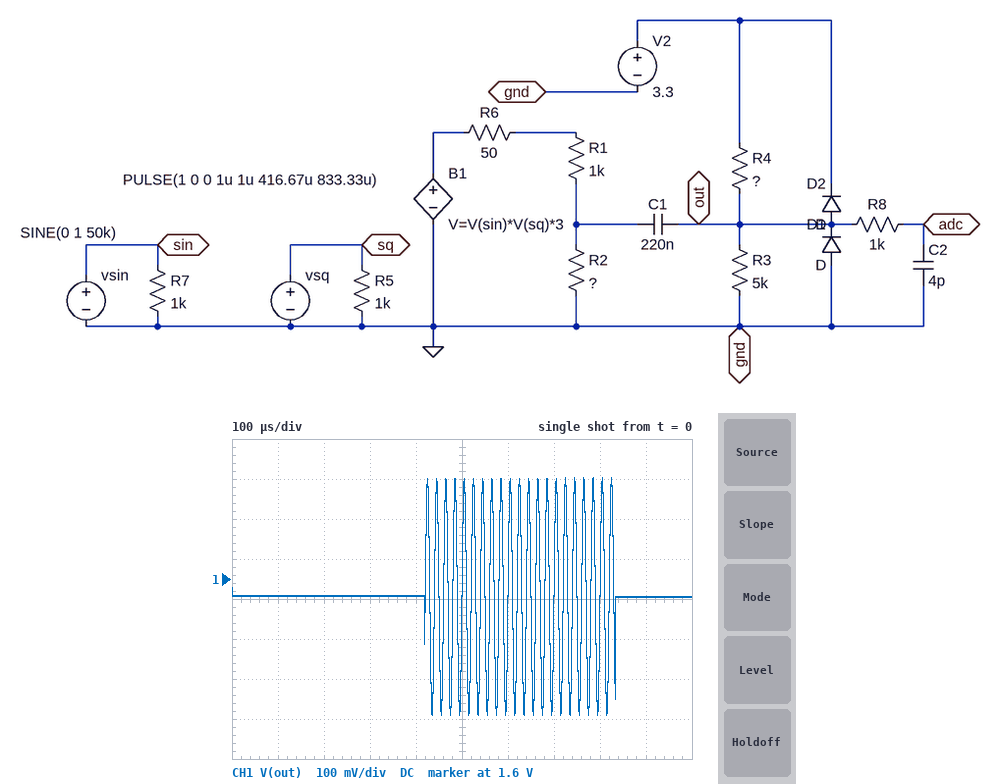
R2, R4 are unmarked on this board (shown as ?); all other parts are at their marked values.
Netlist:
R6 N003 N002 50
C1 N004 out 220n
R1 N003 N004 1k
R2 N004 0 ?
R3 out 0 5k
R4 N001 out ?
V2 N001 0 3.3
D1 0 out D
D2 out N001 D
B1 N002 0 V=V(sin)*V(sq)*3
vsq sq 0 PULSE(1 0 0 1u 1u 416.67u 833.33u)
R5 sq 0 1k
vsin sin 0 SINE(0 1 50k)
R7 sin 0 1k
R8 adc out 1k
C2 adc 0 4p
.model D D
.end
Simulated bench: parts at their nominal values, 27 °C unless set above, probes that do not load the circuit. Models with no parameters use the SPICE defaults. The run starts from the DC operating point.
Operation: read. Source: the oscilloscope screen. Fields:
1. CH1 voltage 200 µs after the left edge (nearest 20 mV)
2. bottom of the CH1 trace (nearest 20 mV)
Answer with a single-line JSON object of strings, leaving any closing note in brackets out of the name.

{"CH1 voltage 200 µs after the left edge": "1.56 V", "bottom of the CH1 trace": "1.26 V"}
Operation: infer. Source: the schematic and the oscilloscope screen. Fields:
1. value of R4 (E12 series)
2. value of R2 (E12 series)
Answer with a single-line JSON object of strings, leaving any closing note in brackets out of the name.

{"value of R4": "5.6 kΩ", "value of R2": "120 Ω"}
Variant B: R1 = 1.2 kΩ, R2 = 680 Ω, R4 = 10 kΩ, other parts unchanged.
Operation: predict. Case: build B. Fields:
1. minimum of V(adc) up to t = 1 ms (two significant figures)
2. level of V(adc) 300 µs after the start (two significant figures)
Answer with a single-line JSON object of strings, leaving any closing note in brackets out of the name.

{"minimum of V(adc) up to t = 1 ms": "160 mV", "level of V(adc) 300 µs after the start": "1.1 V"}
